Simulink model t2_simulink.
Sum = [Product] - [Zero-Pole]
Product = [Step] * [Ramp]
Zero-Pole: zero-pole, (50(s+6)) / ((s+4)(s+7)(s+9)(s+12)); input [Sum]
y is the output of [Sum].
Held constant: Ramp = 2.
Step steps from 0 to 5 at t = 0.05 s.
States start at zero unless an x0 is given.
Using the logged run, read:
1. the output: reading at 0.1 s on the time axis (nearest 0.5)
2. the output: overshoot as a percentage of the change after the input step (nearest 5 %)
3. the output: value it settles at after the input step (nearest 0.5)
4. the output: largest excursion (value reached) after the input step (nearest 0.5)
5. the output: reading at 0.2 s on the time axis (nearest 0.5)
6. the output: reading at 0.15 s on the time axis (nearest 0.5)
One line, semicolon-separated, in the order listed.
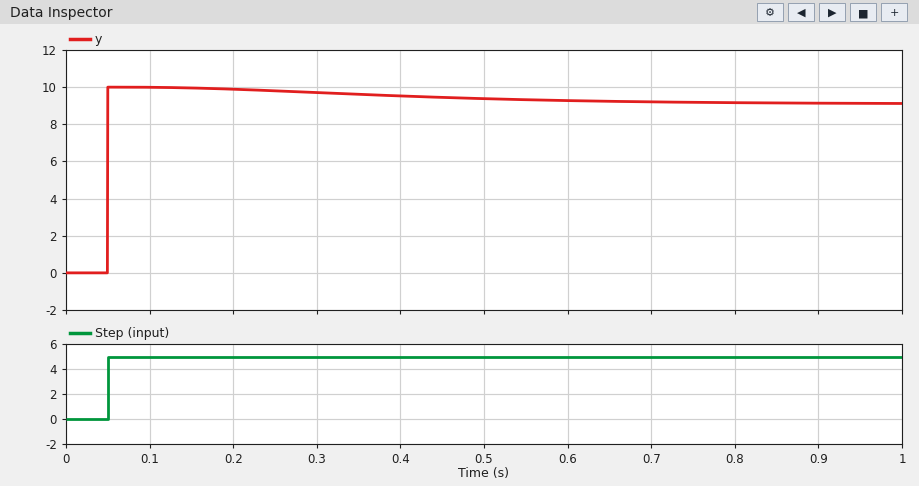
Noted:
10.0; 10 %; 9.0; 10.0; 10.0; 10.0
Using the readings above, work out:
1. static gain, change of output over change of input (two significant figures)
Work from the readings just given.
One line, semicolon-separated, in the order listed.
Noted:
1.8
